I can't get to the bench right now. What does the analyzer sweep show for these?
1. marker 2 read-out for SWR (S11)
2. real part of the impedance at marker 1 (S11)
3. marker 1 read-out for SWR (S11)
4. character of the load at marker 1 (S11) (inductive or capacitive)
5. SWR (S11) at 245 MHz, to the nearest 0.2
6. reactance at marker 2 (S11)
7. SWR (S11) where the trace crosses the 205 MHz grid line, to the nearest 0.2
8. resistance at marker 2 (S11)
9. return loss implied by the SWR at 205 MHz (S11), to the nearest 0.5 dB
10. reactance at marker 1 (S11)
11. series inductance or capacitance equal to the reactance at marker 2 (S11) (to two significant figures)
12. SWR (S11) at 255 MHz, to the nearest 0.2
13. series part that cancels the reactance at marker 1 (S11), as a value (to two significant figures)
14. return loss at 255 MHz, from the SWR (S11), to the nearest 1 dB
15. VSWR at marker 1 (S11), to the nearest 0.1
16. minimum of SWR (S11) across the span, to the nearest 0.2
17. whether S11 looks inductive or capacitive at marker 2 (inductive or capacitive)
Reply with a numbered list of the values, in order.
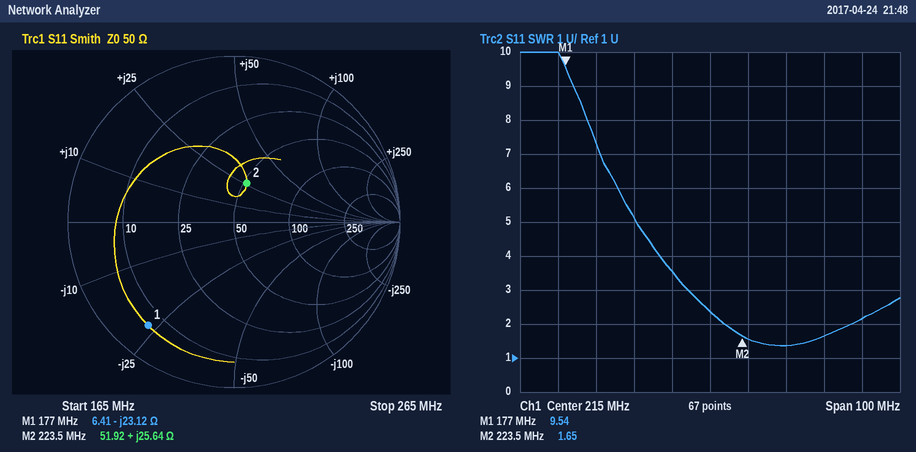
1. 1.65
2. 6.41 Ω
3. 9.54
4. capacitive
5. 1.6
6. +25.64 Ω
7. 3.6
8. 51.92 Ω
9. 5.0 dB
10. -23.12 Ω
11. 18 nH
12. 2.2
13. 21 nH
14. 9 dB
15. 9.5
16. 1.4
17. inductive
